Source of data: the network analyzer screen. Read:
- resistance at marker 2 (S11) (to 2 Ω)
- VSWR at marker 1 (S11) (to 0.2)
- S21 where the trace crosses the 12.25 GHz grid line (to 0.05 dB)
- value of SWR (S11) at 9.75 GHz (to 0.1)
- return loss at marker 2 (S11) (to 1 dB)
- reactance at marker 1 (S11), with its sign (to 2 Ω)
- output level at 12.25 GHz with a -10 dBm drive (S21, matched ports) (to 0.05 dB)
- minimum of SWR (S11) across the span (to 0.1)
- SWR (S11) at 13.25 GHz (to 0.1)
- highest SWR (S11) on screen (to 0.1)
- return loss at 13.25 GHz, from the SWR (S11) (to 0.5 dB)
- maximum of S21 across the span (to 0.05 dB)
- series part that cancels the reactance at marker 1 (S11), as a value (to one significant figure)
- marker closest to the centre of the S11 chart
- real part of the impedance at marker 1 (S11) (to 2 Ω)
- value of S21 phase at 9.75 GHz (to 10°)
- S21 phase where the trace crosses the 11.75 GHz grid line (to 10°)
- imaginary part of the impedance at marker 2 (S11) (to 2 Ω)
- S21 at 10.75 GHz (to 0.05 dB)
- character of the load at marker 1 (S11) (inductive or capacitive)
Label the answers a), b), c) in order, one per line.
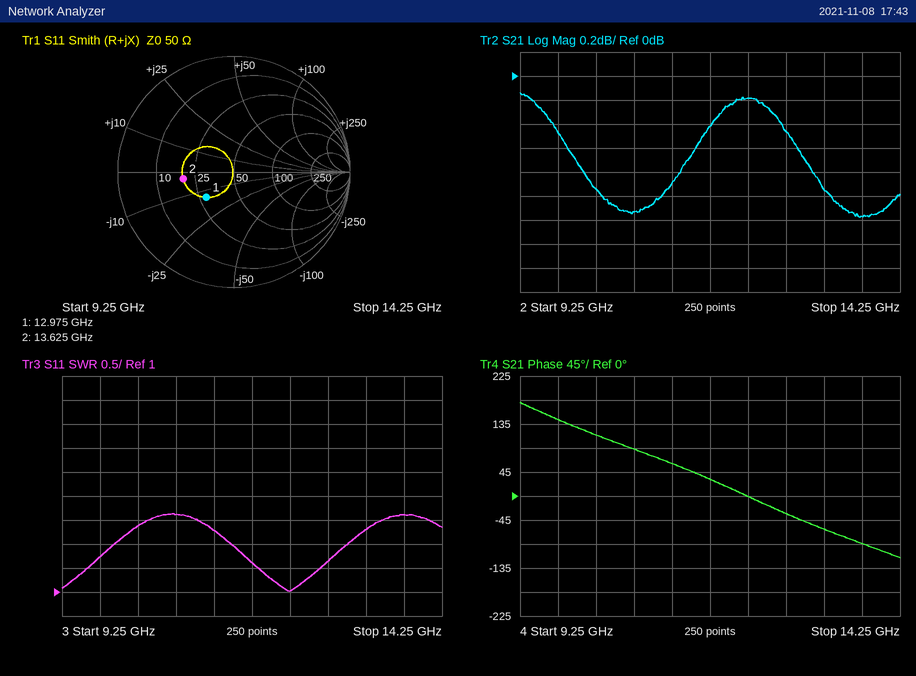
a) 20 Ω
b) 2.0
c) -0.20 dB
d) 1.7
e) 7 dB
f) -14 Ω
g) -10.20 dBm
h) 1.0
i) 2.3
j) 2.6
k) 8.0 dB
l) -0.15 dB
m) 200 pH
n) marker 1
o) 28 Ω
p) 140°
q) 30°
r) -2 Ω
s) -1.15 dB
t) capacitive
